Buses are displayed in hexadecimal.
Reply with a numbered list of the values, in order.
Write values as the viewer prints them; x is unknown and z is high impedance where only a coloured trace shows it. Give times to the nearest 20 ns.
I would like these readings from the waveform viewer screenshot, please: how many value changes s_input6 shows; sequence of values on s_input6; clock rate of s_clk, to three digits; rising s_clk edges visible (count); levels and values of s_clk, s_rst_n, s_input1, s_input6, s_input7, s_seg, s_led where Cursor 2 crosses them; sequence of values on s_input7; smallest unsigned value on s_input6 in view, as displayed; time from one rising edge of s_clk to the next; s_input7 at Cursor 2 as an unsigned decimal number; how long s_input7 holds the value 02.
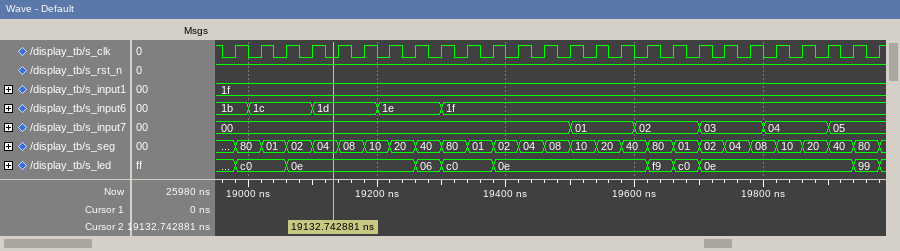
1. 4
2. 1b, 1c, 1d, 1e, 1f
3. 25.0 MHz
4. 26
5. s_clk=0, s_rst_n=1, s_input1=1f, s_input6=1d, s_input7=00, s_seg=04, s_led=0e
6. 00, 01, 02, 03, 04, 05
7. 1b
8. 40 ns
9. 0
10. 100 ns
